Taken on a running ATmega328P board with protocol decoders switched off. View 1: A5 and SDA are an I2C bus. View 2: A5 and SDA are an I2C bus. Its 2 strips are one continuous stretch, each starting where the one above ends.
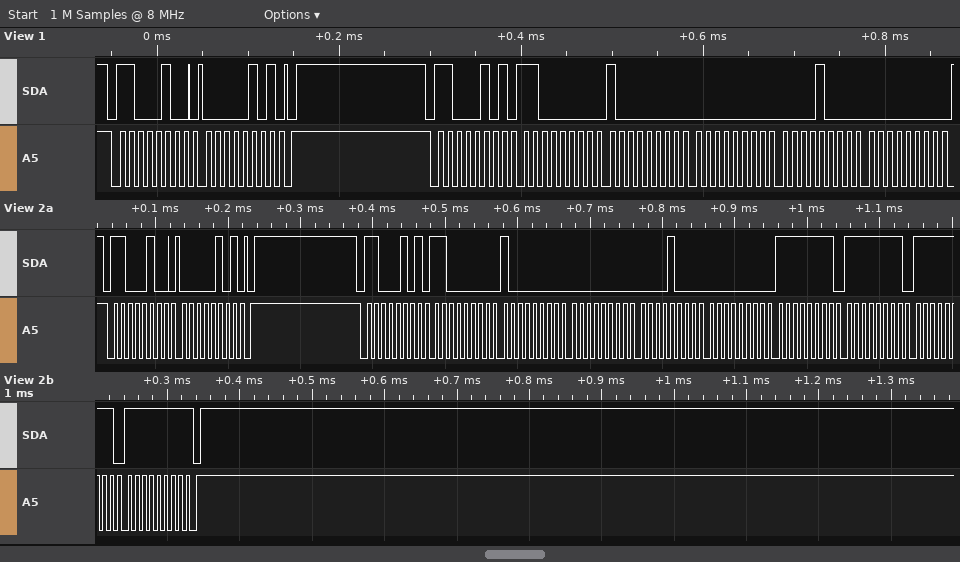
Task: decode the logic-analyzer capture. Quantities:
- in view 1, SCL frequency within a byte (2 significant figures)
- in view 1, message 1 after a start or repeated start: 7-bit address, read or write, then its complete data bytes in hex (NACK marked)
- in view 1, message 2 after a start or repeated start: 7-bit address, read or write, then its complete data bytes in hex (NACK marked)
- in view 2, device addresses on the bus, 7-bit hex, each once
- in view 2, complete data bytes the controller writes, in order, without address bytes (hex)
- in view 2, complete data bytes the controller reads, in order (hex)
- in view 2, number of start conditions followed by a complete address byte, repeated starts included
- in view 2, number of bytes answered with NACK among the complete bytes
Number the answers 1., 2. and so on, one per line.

1. 100 kHz
2. 0x62 write: 05
3. 0x62 read: C0 80 00 08 00
4. 0x62
5. 05
6. C0 80 00 08 00 FF FF FF FF
7. 2
8. 1
